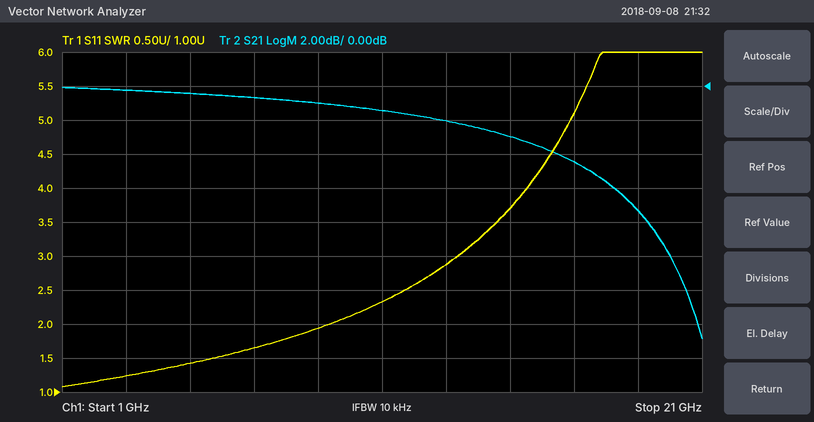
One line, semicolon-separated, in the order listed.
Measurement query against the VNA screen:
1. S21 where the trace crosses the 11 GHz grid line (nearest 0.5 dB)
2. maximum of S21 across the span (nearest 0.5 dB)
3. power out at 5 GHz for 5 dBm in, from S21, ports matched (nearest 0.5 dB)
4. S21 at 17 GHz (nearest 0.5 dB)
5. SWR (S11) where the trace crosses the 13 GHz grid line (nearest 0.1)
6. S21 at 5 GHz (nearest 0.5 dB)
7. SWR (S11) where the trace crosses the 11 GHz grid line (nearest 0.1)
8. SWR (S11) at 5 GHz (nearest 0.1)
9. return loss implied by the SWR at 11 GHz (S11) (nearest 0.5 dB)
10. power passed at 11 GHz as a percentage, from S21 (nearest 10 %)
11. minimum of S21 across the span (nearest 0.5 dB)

-1.5 dB; 0.0 dB; 4.5 dBm; -4.5 dB; 2.9; -0.5 dB; 2.3; 1.4; 8.0 dB; 70 %; -15.0 dB
